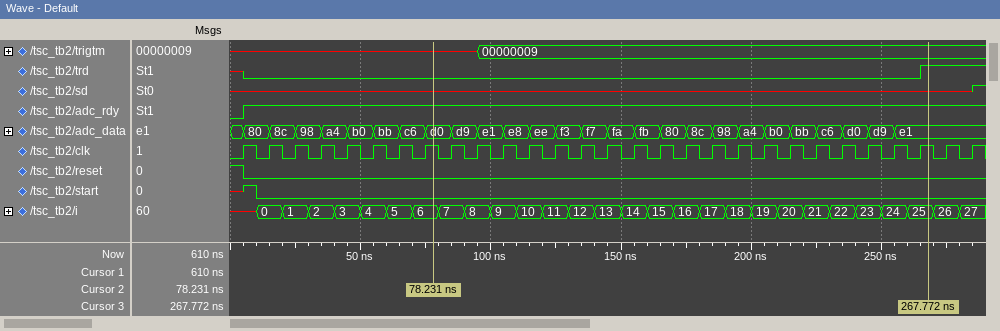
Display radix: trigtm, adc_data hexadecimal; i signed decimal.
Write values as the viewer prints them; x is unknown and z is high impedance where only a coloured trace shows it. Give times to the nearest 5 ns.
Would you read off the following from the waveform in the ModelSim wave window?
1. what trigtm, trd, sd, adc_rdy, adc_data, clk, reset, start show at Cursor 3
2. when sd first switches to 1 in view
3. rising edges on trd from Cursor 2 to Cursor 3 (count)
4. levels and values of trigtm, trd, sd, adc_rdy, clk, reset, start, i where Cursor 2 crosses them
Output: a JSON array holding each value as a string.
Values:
["trigtm=00000009, trd=1, sd=x, adc_rdy=1, adc_data=e1, clk=1, reset=0, start=0", "285 ns", "1", "trigtm=x, trd=0, sd=x, adc_rdy=1, clk=1, reset=0, start=0, i=6"]
